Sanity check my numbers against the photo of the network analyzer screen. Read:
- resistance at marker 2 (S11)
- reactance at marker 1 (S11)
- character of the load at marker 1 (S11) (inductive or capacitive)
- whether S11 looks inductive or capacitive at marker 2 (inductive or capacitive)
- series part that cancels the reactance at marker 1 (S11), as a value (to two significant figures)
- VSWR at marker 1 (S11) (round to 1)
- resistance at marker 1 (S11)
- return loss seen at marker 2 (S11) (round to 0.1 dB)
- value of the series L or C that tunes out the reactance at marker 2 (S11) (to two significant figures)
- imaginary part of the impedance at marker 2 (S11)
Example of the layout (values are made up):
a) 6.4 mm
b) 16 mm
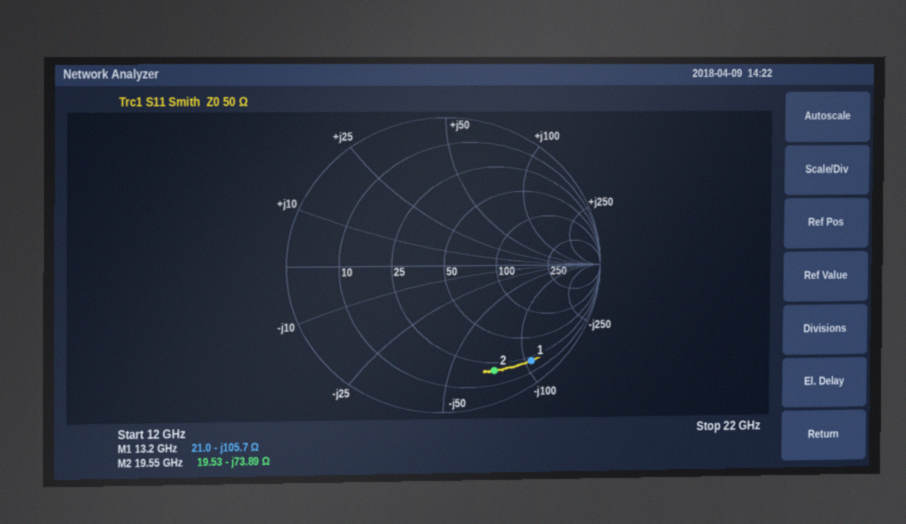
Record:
a) 19.53 Ω
b) -105.7 Ω
c) capacitive
d) capacitive
e) 1.3 nH
f) 13
g) 21.0 Ω
h) 2.1 dB
i) 600 pH
j) -73.89 Ω
